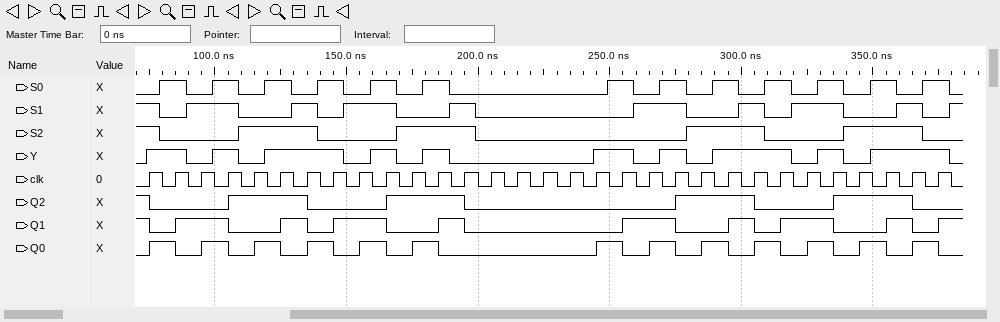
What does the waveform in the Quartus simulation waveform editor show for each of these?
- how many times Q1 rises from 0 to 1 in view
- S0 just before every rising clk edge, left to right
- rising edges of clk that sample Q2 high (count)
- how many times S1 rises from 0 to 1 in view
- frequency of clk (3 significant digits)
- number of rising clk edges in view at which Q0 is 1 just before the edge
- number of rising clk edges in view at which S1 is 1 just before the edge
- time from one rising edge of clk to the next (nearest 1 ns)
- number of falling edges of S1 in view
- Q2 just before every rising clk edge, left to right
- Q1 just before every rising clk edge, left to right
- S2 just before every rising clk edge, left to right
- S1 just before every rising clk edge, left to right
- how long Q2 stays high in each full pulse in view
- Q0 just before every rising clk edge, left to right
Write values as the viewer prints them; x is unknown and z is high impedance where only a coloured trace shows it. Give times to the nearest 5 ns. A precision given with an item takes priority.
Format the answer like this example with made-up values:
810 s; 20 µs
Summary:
9; 0 1 0 1 0 1 0 1 0 1 0 1 0 0 0 0 0 0 1 0 1 0 1 0 1 0 1 0 1 0 1; 13; 9; 100 MHz; 13; 13; 10 ns; 9; 1 0 0 0 1 1 1 0 0 0 1 1 1 0 0 0 0 0 0 0 0 1 1 1 0 0 0 1 1 1 0; 1 0 1 1 0 0 1 0 1 1 0 0 1 0 0 0 0 0 0 1 1 0 0 1 0 1 1 0 0 1 0; 1 0 0 0 1 1 1 0 0 0 1 1 1 0 0 0 0 0 0 0 0 1 1 1 0 0 0 1 1 1 0; 1 0 1 1 0 0 1 0 1 1 0 0 1 0 0 0 0 0 0 1 1 0 0 1 0 1 1 0 0 1 0; 30 ns, 30 ns, 30 ns, 30 ns; 0 1 0 1 0 1 0 1 0 1 0 1 0 0 0 0 0 0 1 0 1 0 1 0 1 0 1 0 1 0 1
